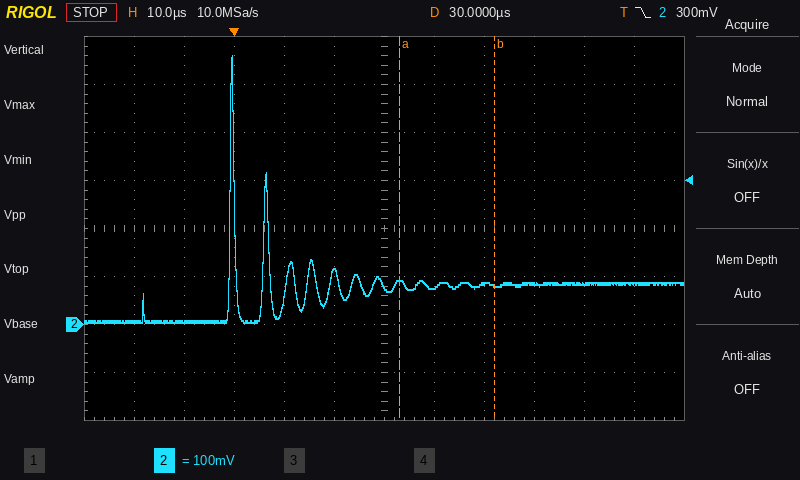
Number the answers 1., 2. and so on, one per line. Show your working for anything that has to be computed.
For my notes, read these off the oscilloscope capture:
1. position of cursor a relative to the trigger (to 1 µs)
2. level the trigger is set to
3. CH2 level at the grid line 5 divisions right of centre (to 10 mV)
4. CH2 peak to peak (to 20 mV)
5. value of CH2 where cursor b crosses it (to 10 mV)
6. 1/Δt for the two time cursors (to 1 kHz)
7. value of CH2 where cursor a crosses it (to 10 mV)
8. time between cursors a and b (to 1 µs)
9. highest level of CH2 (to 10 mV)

1. +33 µs
2. 300 mV
3. 90 mV
4. 560 mV
5. 80 mV
6. 1 / 19 µs ≈ 53 kHz
7. 90 mV
8. 19 µs
9. 560 mV
